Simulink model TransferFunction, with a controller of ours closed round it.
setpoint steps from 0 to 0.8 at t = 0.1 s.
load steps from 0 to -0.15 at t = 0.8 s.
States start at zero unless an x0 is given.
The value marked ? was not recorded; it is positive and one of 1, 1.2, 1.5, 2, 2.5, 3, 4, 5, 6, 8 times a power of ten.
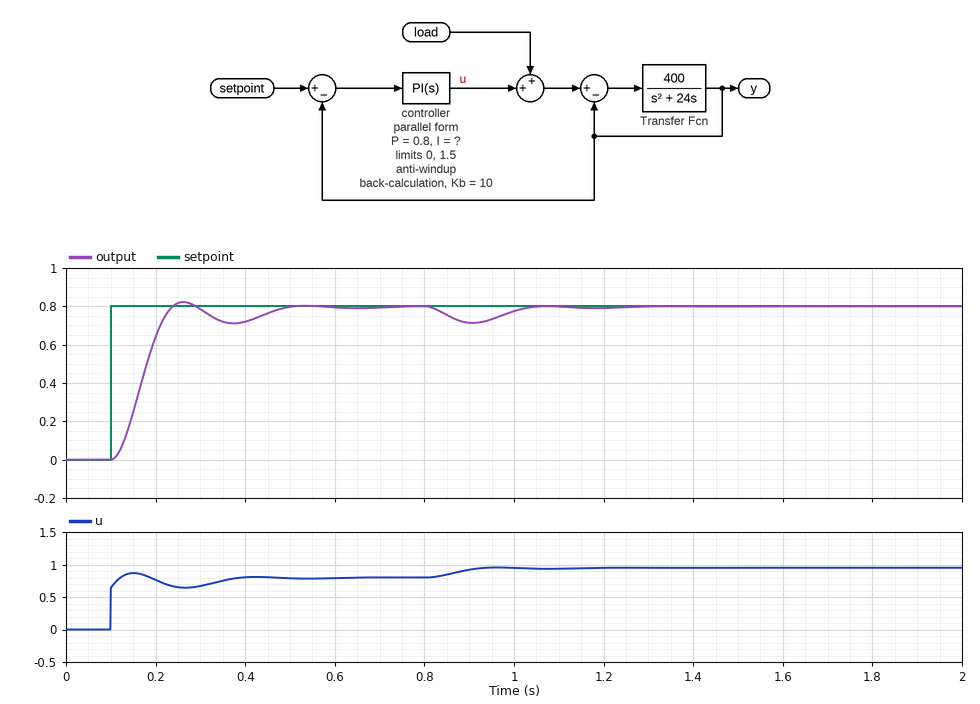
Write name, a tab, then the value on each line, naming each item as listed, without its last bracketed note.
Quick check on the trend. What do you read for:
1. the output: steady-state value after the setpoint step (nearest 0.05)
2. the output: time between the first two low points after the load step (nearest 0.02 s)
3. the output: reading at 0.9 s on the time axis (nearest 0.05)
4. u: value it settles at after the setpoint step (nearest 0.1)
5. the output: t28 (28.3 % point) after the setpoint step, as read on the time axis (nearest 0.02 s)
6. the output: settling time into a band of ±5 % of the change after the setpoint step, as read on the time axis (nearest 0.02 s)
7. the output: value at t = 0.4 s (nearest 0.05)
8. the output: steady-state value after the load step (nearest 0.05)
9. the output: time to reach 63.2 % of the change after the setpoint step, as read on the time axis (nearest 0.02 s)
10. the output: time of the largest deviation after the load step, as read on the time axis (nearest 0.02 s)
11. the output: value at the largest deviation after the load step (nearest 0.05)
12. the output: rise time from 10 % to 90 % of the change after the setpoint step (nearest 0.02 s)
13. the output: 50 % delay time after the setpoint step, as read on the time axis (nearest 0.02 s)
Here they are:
the output: steady-state value after the setpoint step	0.80
the output: time between the first two low points after the load step	0.28 s
the output: reading at 0.9 s on the time axis	0.70
u: value it settles at after the setpoint step	0.8
the output: t28 (28.3 % point) after the setpoint step, as read on the time axis	0.14 s
the output: settling time into a band of ±5 % of the change after the setpoint step, as read on the time axis	0.44 s
the output: value at t = 0.4 s	0.70
the output: steady-state value after the load step	0.80
the output: time to reach 63.2 % of the change after the setpoint step, as read on the time axis	0.18 s
the output: time of the largest deviation after the load step, as read on the time axis	0.90 s
the output: value at the largest deviation after the load step	0.70
the output: rise time from 10 % to 90 % of the change after the setpoint step	0.08 s
the output: 50 % delay time after the setpoint step, as read on the time axis	0.16 s
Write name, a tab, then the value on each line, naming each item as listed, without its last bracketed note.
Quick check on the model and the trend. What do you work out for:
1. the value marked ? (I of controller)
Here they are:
the value marked ?	12
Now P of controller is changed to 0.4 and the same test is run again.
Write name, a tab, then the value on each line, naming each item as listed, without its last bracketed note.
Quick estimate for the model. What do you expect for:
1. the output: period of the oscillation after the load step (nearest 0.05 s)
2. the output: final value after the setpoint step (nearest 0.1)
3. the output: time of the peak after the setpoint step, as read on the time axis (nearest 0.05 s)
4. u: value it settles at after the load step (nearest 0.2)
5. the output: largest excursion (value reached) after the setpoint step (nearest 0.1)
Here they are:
the output: period of the oscillation after the load step	0.35 s
the output: final value after the setpoint step	0.8
the output: time of the peak after the setpoint step, as read on the time axis	0.30 s
u: value it settles at after the load step	1.0
the output: largest excursion (value reached) after the setpoint step	0.9
